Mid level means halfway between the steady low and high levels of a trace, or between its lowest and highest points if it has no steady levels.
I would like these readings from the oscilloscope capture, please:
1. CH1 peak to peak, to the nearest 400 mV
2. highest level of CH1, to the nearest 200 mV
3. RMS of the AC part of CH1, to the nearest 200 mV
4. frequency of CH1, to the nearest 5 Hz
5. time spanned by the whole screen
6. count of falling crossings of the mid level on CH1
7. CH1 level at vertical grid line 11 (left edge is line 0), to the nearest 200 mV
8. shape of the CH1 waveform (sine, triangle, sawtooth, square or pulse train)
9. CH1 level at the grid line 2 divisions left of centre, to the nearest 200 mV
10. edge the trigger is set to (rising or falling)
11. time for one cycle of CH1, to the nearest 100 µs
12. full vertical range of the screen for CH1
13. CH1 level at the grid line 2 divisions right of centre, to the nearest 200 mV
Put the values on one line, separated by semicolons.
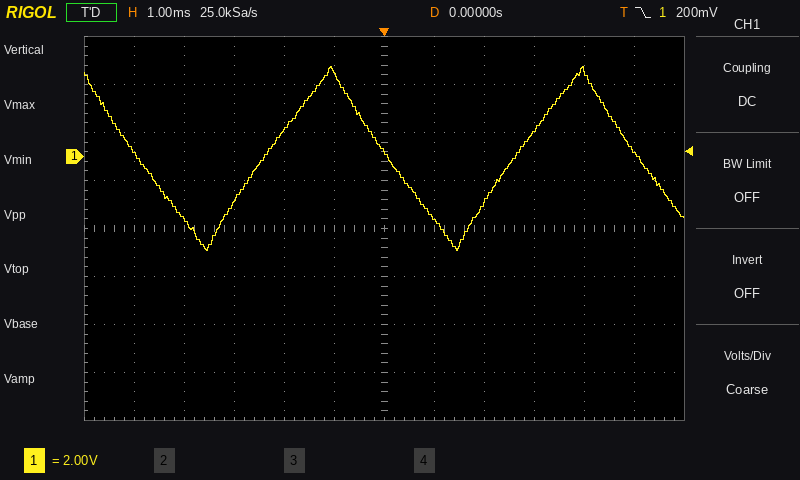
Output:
7.6 V; 3.8 V; 2.2 V; 200 Hz; 12 ms; 3; 200 mV; triangle; 1.0 V; falling; 5.0 ms; 16 V; -2.0 V
